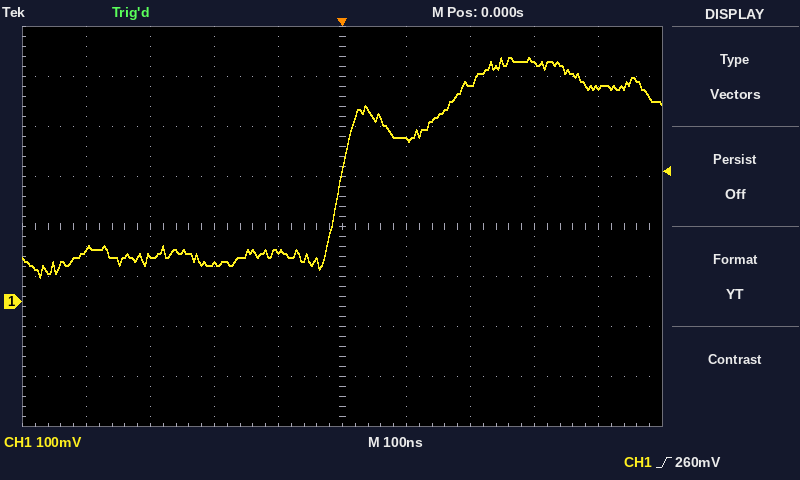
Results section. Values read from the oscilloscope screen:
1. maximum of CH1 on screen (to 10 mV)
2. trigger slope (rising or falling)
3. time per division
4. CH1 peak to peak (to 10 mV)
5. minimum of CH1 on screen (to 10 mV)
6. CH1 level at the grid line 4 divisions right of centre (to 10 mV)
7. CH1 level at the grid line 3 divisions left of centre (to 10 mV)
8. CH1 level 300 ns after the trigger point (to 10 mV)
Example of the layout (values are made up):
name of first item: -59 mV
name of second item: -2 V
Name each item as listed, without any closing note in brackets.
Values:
maximum of CH1 on screen: 490 mV
trigger slope: rising
time per division: 100 ns
CH1 peak to peak: 440 mV
minimum of CH1 on screen: 50 mV
CH1 level at the grid line 4 divisions right of centre: 430 mV
CH1 level at the grid line 3 divisions left of centre: 90 mV
CH1 level 300 ns after the trigger point: 480 mV
